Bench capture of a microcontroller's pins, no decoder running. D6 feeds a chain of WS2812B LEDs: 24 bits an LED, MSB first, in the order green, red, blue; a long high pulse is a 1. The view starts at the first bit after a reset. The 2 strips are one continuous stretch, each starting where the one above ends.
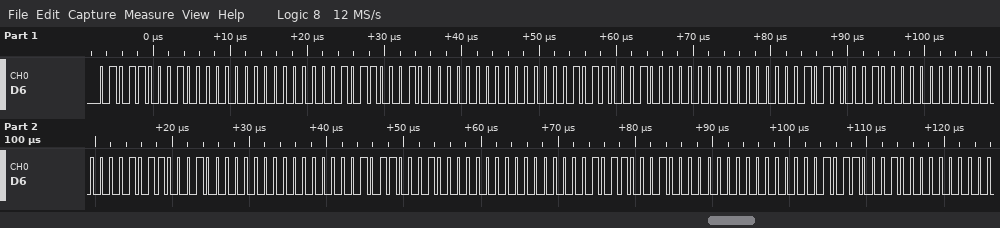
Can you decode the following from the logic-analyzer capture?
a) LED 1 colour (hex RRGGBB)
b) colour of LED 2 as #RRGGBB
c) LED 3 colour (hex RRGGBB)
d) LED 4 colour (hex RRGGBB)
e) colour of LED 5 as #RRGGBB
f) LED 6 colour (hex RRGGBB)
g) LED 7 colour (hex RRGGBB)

#805800
#805800
#805800
#805800
#805800
#805800
#805800
